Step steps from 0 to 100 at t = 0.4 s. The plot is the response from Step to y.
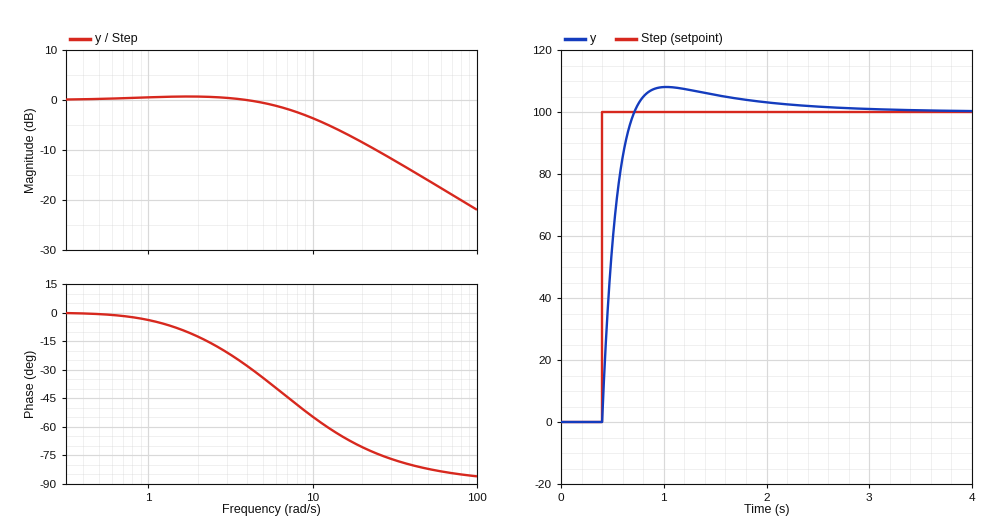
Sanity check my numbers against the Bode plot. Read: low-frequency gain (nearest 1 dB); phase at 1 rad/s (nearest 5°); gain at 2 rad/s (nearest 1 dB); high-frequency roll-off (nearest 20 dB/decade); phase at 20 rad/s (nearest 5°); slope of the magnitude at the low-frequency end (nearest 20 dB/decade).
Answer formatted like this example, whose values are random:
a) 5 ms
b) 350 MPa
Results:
a) 0 dB
b) -5°
c) 1 dB
d) -20 dB/decade
e) -70°
f) 0 dB/decade
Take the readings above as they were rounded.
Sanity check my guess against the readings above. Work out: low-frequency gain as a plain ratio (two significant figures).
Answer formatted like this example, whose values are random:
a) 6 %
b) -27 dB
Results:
a) 1.0
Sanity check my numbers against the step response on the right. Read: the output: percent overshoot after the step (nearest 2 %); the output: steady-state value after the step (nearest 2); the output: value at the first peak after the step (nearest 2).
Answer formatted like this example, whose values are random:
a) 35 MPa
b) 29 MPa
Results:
a) 8 %
b) 100
c) 108
